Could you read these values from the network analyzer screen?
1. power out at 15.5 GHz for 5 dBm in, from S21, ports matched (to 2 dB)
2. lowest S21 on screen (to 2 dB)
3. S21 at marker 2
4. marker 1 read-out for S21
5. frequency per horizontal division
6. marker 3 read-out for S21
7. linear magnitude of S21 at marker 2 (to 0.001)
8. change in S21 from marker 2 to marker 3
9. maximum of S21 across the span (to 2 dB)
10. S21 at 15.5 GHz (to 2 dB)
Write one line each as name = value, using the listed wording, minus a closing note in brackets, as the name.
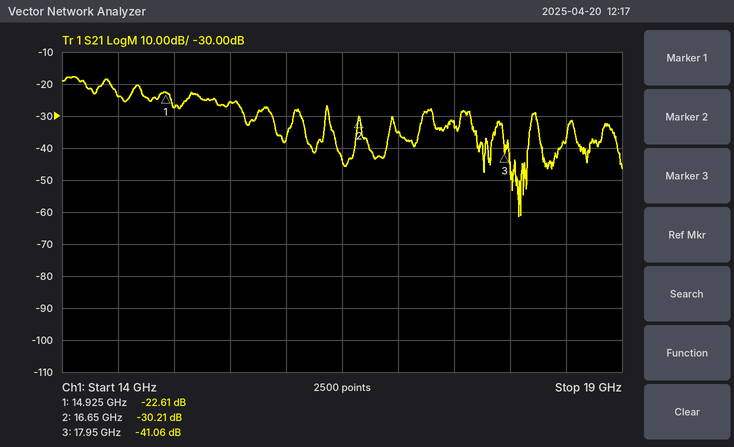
power out at 15.5 GHz for 5 dBm in, from S21, ports matched = -20 dBm
lowest S21 on screen = -62 dB
S21 at marker 2 = -30.21 dB
marker 1 read-out for S21 = -22.61 dB
frequency per horizontal division = 500 MHz
marker 3 read-out for S21 = -41.06 dB
linear magnitude of S21 at marker 2 = 0.031
change in S21 from marker 2 to marker 3 = -10.85 dB
maximum of S21 across the span = -18 dB
S21 at 15.5 GHz = -26 dB
